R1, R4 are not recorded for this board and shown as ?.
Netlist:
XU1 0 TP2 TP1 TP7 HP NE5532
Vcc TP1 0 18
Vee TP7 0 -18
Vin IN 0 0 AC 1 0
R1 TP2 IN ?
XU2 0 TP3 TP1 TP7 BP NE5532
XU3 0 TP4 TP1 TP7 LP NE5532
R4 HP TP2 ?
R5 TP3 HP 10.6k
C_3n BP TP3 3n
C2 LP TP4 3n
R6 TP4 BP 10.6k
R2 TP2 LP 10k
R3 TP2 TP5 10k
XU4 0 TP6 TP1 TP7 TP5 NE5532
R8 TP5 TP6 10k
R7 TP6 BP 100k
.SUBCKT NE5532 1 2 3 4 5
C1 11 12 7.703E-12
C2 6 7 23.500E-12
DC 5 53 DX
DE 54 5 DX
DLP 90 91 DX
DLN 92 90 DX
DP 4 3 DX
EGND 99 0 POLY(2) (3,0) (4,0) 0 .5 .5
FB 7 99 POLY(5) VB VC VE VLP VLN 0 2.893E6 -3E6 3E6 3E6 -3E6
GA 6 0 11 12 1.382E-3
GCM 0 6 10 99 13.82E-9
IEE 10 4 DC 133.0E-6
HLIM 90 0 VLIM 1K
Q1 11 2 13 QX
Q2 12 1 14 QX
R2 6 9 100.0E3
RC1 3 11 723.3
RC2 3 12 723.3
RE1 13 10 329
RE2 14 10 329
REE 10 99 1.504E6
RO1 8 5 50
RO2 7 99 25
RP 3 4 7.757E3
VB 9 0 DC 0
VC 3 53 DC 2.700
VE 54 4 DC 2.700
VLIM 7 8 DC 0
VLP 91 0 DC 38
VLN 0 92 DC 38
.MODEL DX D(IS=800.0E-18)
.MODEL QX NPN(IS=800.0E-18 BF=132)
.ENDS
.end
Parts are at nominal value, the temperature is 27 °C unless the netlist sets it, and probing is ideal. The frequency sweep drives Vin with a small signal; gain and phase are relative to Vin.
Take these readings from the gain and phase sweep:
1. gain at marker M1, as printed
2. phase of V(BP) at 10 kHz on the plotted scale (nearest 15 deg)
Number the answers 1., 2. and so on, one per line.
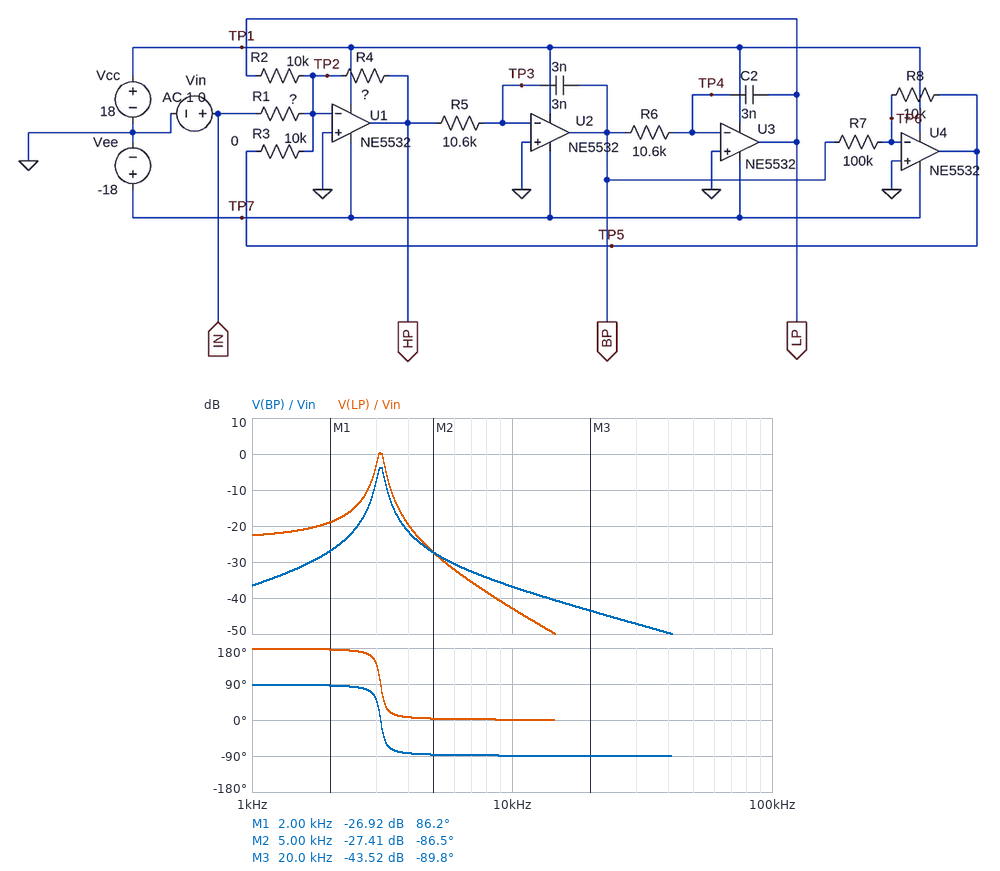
1. -26.92 dB
2. -90 deg
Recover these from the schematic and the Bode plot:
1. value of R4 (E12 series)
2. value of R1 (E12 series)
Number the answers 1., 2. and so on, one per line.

1. 3.9 kΩ
2. 150 kΩ
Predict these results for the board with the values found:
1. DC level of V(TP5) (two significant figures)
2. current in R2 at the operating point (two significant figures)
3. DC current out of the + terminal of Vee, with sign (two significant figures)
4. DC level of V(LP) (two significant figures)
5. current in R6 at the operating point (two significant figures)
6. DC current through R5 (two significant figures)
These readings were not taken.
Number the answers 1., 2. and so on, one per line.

1. 4.5 mV
2. 1.3 µA
3. -19 mA
4. -13 mV
5. 500 nA
6. 500 nA
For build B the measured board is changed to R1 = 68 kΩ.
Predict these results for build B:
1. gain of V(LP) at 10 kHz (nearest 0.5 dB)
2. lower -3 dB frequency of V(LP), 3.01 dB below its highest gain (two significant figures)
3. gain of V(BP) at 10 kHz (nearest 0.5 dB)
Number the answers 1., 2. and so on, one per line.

1. -36.0 dB
2. 3.0 kHz
3. -30.0 dB
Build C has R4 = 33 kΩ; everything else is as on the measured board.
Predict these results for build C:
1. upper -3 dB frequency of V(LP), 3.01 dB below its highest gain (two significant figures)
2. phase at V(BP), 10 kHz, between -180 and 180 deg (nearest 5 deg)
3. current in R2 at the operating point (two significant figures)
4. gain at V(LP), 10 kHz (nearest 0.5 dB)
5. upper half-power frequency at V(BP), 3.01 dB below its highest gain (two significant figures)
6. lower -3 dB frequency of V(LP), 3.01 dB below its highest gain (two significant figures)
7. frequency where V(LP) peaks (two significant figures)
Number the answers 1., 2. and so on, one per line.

1. 9.8 kHz
2. -50 deg
3. 110 nA
4. -12.5 dB
5. 9.9 kHz
6. 8.2 kHz
7. 9.0 kHz
